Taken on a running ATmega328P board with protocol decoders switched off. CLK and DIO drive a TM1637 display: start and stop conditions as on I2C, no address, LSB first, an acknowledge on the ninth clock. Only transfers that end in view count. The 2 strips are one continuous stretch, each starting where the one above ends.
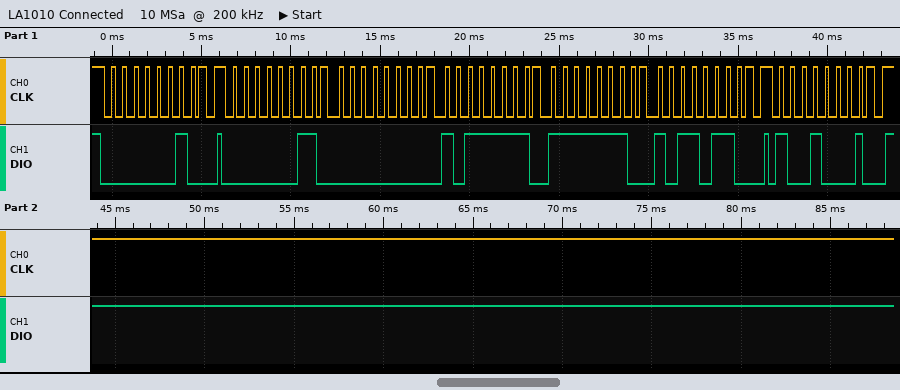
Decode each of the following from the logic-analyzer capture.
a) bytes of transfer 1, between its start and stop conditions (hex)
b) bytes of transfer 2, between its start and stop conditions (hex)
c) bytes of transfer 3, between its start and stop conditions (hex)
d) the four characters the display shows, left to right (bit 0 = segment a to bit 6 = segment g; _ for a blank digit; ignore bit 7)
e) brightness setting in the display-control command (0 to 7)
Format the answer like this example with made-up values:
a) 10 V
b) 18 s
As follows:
a) 40
b) C0 00 FD 7F 6D
c) 89
d) _685
e) 1
